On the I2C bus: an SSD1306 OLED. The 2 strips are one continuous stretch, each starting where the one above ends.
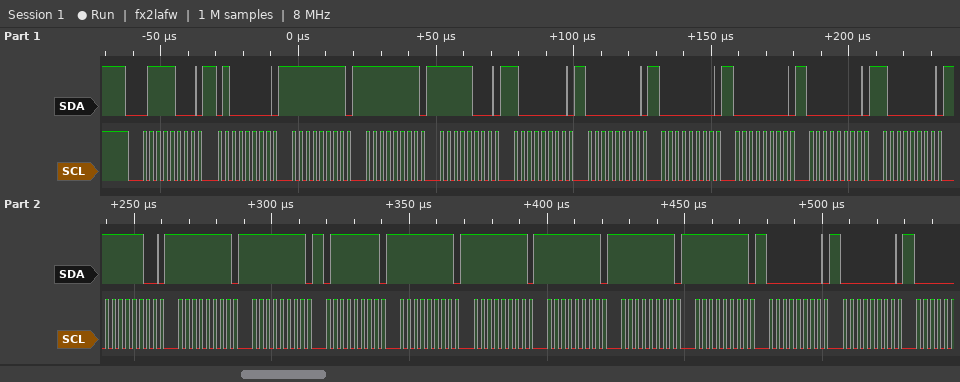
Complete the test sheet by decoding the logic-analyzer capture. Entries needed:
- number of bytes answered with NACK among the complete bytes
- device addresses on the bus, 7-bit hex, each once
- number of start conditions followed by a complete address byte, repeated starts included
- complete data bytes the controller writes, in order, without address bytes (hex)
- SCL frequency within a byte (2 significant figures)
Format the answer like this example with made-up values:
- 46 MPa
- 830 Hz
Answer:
- 0
- 0x3C
- 1
- 40 FF FF F8 80 00 00 00 00 80 FC FF FF 7F FF FF FF FF FF 00 00
- 400 kHz
